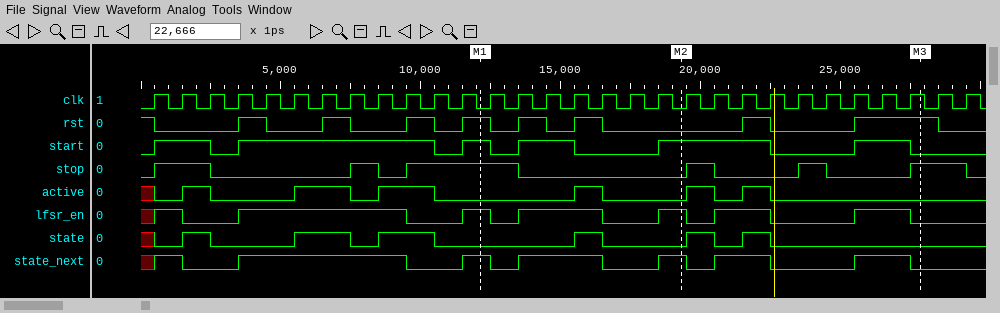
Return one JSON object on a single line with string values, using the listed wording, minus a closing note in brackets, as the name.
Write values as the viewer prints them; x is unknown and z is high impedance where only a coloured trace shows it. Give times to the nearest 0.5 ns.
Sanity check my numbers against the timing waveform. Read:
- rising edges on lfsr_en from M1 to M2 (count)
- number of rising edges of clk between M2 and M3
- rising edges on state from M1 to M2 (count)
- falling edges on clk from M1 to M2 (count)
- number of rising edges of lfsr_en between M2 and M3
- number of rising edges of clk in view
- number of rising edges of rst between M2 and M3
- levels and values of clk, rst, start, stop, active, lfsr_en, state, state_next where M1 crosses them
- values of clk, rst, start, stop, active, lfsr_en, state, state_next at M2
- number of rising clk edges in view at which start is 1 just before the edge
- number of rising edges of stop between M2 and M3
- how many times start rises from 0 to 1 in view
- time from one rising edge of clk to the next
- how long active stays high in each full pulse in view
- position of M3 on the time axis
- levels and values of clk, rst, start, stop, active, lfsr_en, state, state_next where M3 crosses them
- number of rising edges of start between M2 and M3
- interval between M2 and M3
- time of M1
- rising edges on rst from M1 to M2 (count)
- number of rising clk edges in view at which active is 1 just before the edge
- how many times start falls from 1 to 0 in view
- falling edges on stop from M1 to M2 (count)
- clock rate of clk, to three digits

{"rising edges on lfsr_en from M1 to M2": "2", "number of rising edges of clk between M2 and M3": "9", "rising edges on state from M1 to M2": "1", "falling edges on clk from M1 to M2": "7", "number of rising edges of lfsr_en between M2 and M3": "2", "number of rising edges of clk in view": "30", "number of rising edges of rst between M2 and M3": "2", "levels and values of clk, rst, start, stop, active, lfsr_en, state, state_next where M1 crosses them": "clk=0, rst=1, start=1, stop=1, active=0, lfsr_en=1, state=0, state_next=1", "values of clk, rst, start, stop, active, lfsr_en, state, state_next at M2": "clk=0, rst=0, start=1, stop=0, active=0, lfsr_en=1, state=0, state_next=1", "number of rising clk edges in view at which start is 1 just before the edge": "18", "number of rising edges of stop between M2 and M3": "3", "how many times start rises from 0 to 1 in view": "6", "time from one rising edge of clk to the next": "1 ns", "how long active stays high in each full pulse in view": "1 ns, 2 ns, 2 ns, 1 ns, 1 ns, 1 ns", "position of M3 on the time axis": "28 ns", "levels and values of clk, rst, start, stop, active, lfsr_en, state, state_next where M3 crosses them": "clk=1, rst=1, start=0, stop=1, active=0, lfsr_en=0, state=0, state_next=0", "number of rising edges of start between M2 and M3": "1", "interval between M2 and M3": "8.5 ns", "time of M1": "12 ns", "rising edges on rst from M1 to M2": "2", "number of rising clk edges in view at which active is 1 just before the edge": "8", "how many times start falls from 1 to 0 in view": "6", "falling edges on stop from M1 to M2": "1", "clock rate of clk, to three digits": "1.00 GHz"}
